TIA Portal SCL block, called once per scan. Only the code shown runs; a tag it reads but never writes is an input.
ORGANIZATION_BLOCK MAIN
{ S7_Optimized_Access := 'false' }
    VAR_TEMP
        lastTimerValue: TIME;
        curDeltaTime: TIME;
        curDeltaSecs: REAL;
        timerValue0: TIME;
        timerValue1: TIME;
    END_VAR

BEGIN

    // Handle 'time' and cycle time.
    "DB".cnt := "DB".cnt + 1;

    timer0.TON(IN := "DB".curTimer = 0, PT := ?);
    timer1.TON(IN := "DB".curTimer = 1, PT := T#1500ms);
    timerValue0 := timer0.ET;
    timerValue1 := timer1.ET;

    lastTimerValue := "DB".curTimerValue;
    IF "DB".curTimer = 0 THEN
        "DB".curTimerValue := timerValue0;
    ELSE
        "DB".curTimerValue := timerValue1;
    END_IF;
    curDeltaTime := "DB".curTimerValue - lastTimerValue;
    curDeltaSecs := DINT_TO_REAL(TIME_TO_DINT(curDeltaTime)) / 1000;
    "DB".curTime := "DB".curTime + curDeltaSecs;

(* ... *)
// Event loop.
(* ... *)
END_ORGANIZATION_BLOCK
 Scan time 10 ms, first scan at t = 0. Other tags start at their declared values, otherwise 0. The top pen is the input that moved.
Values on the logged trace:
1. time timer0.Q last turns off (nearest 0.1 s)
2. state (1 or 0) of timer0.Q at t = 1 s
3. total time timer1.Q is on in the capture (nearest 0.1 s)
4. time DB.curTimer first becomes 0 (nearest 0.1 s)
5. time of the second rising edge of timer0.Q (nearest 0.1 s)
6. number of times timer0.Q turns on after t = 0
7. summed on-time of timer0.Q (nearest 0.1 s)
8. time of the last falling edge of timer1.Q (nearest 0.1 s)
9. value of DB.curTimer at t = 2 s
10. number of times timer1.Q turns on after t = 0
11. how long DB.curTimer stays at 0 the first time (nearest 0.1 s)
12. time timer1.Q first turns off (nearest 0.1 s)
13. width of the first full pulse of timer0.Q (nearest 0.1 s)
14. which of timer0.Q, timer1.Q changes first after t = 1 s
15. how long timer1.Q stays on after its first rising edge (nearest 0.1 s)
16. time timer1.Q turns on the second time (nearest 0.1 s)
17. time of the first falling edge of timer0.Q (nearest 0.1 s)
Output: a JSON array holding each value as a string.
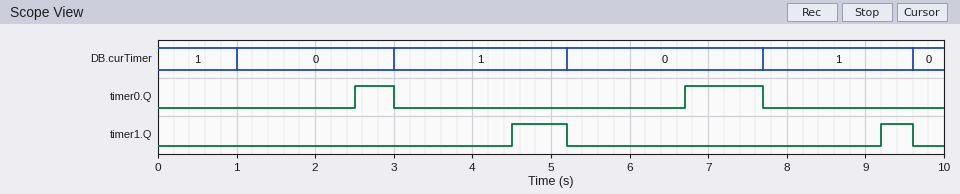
["7.7 s", "0", "1.1 s", "1.0 s", "6.7 s", "2", "1.5 s", "9.6 s", "0", "2", "2.0 s", "5.2 s", "0.5 s", "timer0.Q", "0.7 s", "9.2 s", "3.0 s"]
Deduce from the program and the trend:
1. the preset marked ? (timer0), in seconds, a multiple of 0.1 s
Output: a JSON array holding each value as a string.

["1.5 s"]
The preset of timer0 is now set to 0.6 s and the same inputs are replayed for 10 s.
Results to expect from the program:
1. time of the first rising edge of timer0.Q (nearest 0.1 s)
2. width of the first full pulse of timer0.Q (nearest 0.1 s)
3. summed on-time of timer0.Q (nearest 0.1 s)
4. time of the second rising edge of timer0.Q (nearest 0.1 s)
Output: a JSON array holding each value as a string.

["1.6 s", "1.4 s", "3.3 s", "5.8 s"]
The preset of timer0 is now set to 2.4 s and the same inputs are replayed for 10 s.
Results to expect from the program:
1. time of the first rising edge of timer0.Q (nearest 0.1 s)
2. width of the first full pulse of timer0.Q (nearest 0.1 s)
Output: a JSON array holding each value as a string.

["7.6 s", "0.1 s"]
